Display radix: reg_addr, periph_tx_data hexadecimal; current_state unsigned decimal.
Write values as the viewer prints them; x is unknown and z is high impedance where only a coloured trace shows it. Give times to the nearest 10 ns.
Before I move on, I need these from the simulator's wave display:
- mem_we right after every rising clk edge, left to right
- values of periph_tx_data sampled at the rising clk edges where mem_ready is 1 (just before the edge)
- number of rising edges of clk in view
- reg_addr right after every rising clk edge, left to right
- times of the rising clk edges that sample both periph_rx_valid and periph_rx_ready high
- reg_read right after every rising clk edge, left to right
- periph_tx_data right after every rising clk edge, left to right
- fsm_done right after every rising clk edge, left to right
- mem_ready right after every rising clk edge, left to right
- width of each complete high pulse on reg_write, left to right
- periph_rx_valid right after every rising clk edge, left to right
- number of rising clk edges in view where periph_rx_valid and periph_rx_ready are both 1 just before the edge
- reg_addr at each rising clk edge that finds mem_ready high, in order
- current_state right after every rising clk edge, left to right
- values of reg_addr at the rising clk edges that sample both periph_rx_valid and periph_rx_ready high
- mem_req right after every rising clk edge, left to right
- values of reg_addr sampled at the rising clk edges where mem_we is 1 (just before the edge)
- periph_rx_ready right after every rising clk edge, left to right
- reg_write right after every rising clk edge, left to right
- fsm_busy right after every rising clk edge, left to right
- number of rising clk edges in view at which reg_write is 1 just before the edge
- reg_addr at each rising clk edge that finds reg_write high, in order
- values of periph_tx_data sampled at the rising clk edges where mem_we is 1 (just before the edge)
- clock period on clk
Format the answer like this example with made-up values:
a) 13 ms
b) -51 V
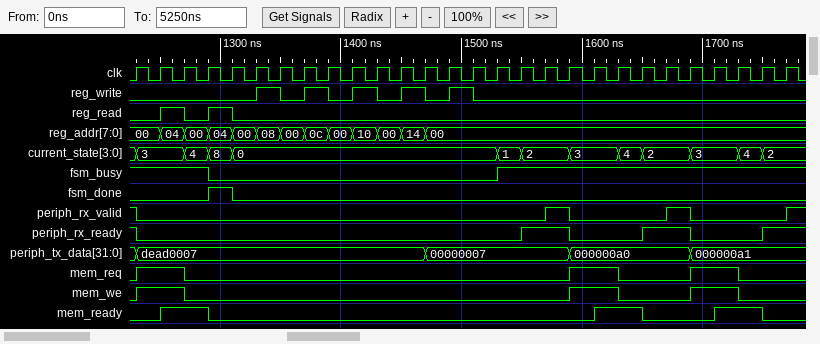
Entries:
a) 1 1 0 0 0 0 0 0 0 0 0 0 0 0 0 0 0 0 1 1 0 0 0 1 1 0 0 0
b) dead0007, dead0007, 000000a0, 000000a0, 000000a1, 000000a1
c) 28
d) 00, 04, 00, 04, 00, 08, 00, 0c, 00, 10, 00, 14, 00, 00, 00, 00, 00, 00, 00, 00, 00, 00, 00, 00, 00, 00, 00, 00
e) 1230 ns, 1590 ns, 1690 ns
f) 0 1 0 1 0 0 0 0 0 0 0 0 0 0 0 0 0 0 0 0 0 0 0 0 0 0 0 0
g) dead0007, dead0007, dead0007, dead0007, dead0007, dead0007, dead0007, dead0007, dead0007, dead0007, dead0007, dead0007, 00000007, 00000007, 00000007, 00000007, 00000007, 00000007, 000000a0, 000000a0, 000000a0, 000000a0, 000000a0, 000000a1, 000000a1, 000000a1, 000000a1, 000000a1
h) 0 0 0 1 0 0 0 0 0 0 0 0 0 0 0 0 0 0 0 0 0 0 0 0 0 0 0 0
i) 0 1 1 0 0 0 0 0 0 0 0 0 0 0 0 0 0 0 0 1 1 0 0 0 1 1 0 0
j) 20 ns, 20 ns, 20 ns, 20 ns, 20 ns
k) 0 0 0 0 0 0 0 0 0 0 0 0 0 0 0 0 0 1 0 0 0 0 1 0 0 0 0 1
l) 3
m) 04, 00, 00, 00, 00, 00
n) 3, 3, 4, 8, 0, 0, 0, 0, 0, 0, 0, 0, 0, 0, 0, 1, 2, 2, 3, 3, 4, 2, 2, 3, 3, 4, 2, 2
o) 00, 00, 00
p) 1 1 0 0 0 0 0 0 0 0 0 0 0 0 0 0 0 0 1 1 0 0 0 1 1 0 0 0
q) 00, 04, 00, 00, 00, 00
r) 0 0 0 0 0 0 0 0 0 0 0 0 0 0 0 0 1 1 0 0 0 1 1 0 0 0 1 1
s) 0 0 0 0 0 1 0 1 0 1 0 1 0 1 0 0 0 0 0 0 0 0 0 0 0 0 0 0
t) 1 1 1 0 0 0 0 0 0 0 0 0 0 0 0 1 1 1 1 1 1 1 1 1 1 1 1 1
u) 5
v) 08, 0c, 10, 14, 00
w) dead0007, dead0007, 000000a0, 000000a0, 000000a1, 000000a1
x) 20 ns
